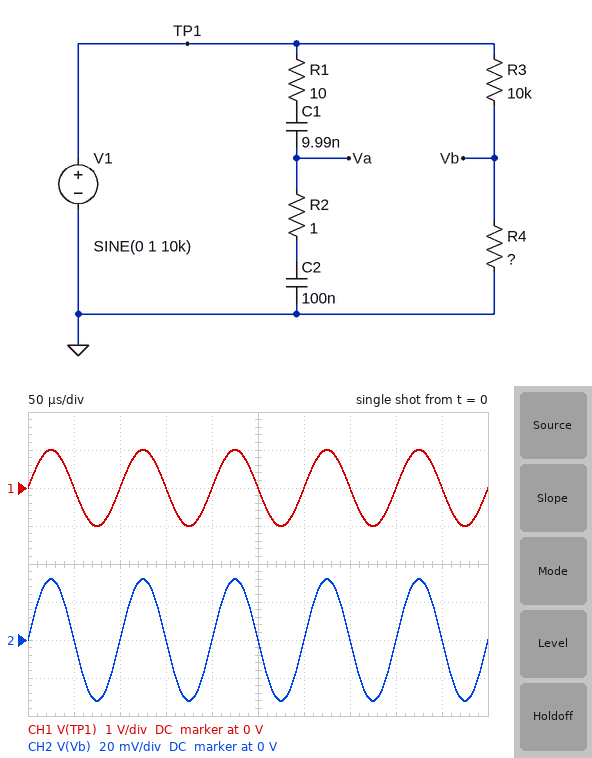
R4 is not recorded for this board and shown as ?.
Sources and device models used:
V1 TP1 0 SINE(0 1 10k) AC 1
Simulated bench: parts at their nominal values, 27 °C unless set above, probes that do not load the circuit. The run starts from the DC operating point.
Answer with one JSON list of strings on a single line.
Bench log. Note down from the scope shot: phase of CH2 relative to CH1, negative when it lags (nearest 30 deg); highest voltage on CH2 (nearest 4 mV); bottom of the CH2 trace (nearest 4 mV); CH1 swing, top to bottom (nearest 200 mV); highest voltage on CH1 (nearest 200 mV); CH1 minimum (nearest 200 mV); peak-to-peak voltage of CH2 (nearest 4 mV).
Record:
["0 deg", "32 mV", "-32 mV", "2.0 V", "1.0 V", "-1.0 V", "64 mV"]
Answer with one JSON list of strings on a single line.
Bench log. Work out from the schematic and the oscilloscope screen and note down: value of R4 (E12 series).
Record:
["330 Ω"]
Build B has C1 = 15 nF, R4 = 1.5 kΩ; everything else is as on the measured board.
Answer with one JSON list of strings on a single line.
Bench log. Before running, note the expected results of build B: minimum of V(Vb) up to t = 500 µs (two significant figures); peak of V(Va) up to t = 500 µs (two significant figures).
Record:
["-130 mV", "130 mV"]
